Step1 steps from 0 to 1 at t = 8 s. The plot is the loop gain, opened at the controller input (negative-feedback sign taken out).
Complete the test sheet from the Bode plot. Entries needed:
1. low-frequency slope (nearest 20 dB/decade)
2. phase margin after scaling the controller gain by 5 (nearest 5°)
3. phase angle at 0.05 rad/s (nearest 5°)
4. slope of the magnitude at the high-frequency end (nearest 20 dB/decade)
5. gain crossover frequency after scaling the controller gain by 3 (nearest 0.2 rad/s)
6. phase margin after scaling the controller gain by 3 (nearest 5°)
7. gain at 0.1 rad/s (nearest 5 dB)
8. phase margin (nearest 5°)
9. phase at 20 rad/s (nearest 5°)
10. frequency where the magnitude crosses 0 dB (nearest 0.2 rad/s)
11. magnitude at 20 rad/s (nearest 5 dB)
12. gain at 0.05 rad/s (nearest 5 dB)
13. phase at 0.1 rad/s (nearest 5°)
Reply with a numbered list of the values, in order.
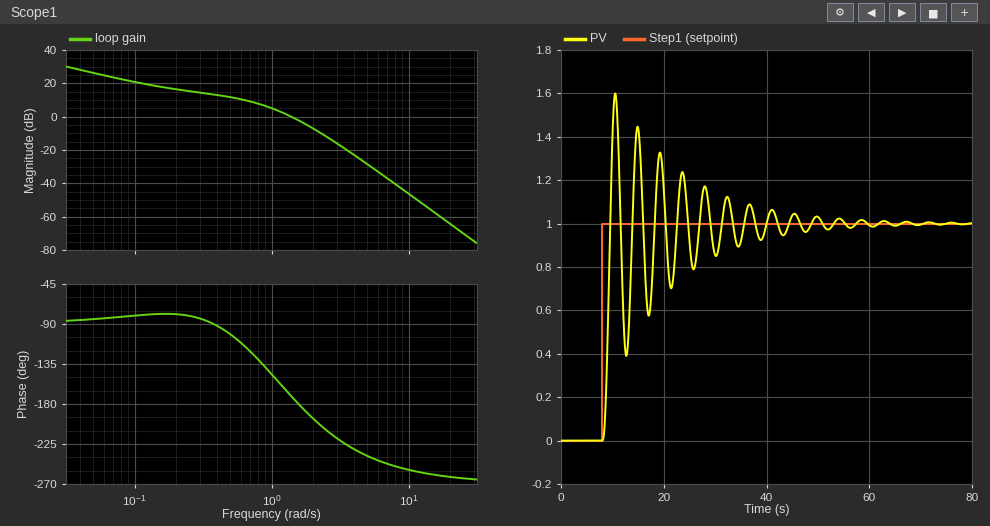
1. -20 dB/decade
2. -35°
3. -85°
4. -60 dB/decade
5. 2.2 rad/s
6. -25°
7. 20 dB
8. 10°
9. -260°
10. 1.4 rad/s
11. -65 dB
12. 25 dB
13. -80°
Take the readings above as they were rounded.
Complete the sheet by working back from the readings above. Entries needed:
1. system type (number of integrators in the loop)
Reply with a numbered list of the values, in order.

1. 1
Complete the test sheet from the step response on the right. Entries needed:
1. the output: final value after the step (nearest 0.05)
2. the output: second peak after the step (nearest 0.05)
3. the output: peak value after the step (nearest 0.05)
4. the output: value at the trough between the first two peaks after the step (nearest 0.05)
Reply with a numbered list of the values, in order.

1. 1.00
2. 1.45
3. 1.60
4. 0.40
